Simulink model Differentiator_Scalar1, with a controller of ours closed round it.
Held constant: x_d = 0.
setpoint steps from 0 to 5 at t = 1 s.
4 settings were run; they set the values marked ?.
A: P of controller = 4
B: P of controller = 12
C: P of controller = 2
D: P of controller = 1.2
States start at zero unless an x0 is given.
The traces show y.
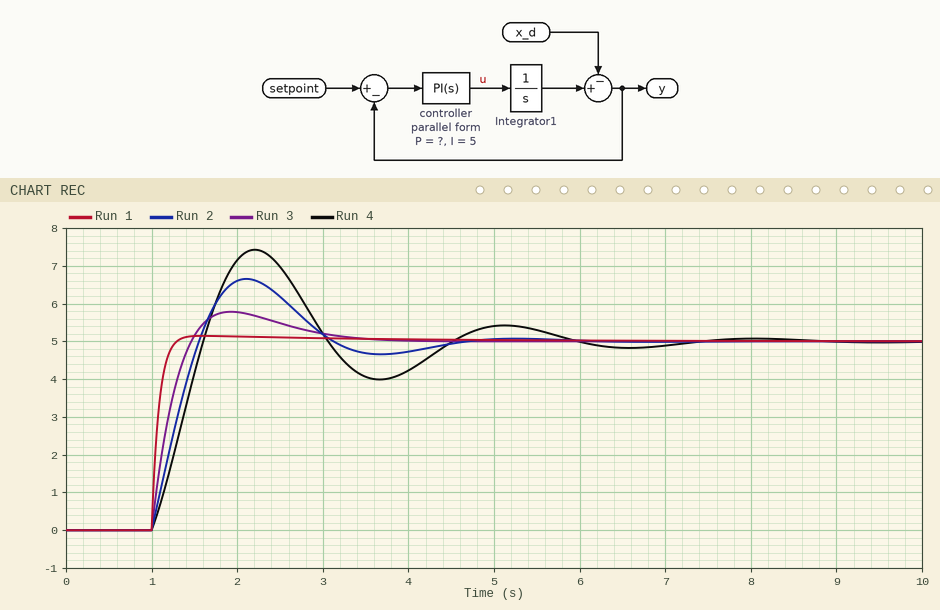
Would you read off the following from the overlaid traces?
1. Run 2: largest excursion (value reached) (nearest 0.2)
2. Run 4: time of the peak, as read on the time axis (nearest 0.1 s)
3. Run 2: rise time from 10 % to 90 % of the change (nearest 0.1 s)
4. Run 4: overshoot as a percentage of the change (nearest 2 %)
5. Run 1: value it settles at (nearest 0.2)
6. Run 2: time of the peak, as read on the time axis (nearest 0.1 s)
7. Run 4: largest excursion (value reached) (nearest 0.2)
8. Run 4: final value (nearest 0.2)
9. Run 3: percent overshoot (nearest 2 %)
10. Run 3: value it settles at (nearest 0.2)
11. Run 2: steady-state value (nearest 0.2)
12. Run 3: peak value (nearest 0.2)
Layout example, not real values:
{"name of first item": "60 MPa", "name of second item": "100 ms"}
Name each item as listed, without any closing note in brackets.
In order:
{"Run 2: largest excursion (value reached)": "6.6", "Run 4: time of the peak, as read on the time axis": "2.2 s", "Run 2: rise time from 10 % to 90 % of the change": "0.4 s", "Run 4: overshoot as a percentage of the change": "48 %", "Run 1: value it settles at": "5.0", "Run 2: time of the peak, as read on the time axis": "2.1 s", "Run 4: largest excursion (value reached)": "7.4", "Run 4: final value": "5.0", "Run 3: percent overshoot": "16 %", "Run 3: value it settles at": "5.0", "Run 2: steady-state value": "5.0", "Run 3: peak value": "5.8"}
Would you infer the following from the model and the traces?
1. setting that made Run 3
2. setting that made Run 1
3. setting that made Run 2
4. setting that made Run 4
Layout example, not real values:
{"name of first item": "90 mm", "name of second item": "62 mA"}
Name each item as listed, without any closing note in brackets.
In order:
{"setting that made Run 3": "A", "setting that made Run 1": "B", "setting that made Run 2": "C", "setting that made Run 4": "D"}
